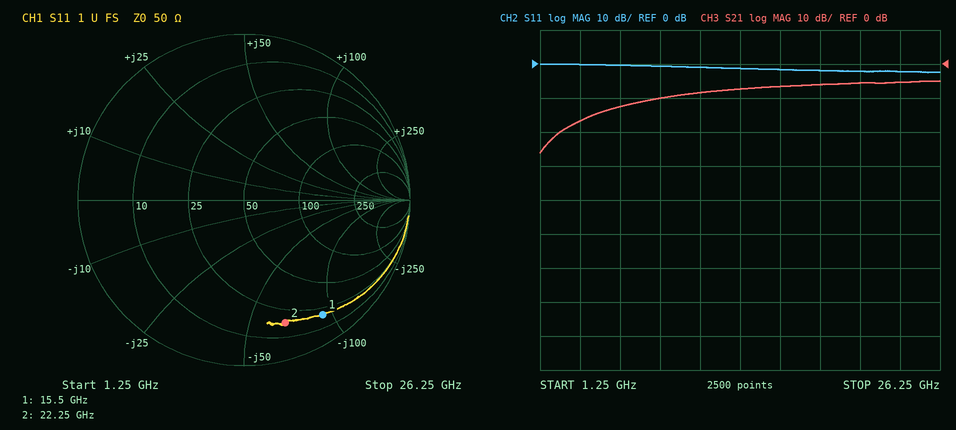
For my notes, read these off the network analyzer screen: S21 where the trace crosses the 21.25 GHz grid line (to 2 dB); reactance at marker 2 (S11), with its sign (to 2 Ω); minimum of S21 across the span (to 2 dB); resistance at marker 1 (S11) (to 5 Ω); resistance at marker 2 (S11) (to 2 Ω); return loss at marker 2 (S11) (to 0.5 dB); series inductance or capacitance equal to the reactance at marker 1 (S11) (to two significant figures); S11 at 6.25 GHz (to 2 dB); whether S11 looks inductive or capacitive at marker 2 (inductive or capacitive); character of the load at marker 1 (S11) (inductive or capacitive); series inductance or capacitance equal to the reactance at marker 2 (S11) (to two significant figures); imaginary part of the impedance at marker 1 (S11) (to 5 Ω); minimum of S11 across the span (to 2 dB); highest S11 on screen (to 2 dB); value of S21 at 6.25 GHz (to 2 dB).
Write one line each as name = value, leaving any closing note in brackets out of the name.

S21 where the trace crosses the 21.25 GHz grid line = -6 dB
reactance at marker 2 (S11), with its sign = -66 Ω
minimum of S21 across the span = -26 dB
resistance at marker 1 (S11) = 20 Ω
resistance at marker 2 (S11) = 18 Ω
return loss at marker 2 (S11) = 2.0 dB
series inductance or capacitance equal to the reactance at marker 1 (S11) = 110 fF
S11 at 6.25 GHz = 0 dB
whether S11 looks inductive or capacitive at marker 2 = capacitive
character of the load at marker 1 (S11) = capacitive
series inductance or capacitance equal to the reactance at marker 2 (S11) = 110 fF
imaginary part of the impedance at marker 1 (S11) = -90 Ω
minimum of S11 across the span = -2 dB
highest S11 on screen = 0 dB
value of S21 at 6.25 GHz = -12 dB
